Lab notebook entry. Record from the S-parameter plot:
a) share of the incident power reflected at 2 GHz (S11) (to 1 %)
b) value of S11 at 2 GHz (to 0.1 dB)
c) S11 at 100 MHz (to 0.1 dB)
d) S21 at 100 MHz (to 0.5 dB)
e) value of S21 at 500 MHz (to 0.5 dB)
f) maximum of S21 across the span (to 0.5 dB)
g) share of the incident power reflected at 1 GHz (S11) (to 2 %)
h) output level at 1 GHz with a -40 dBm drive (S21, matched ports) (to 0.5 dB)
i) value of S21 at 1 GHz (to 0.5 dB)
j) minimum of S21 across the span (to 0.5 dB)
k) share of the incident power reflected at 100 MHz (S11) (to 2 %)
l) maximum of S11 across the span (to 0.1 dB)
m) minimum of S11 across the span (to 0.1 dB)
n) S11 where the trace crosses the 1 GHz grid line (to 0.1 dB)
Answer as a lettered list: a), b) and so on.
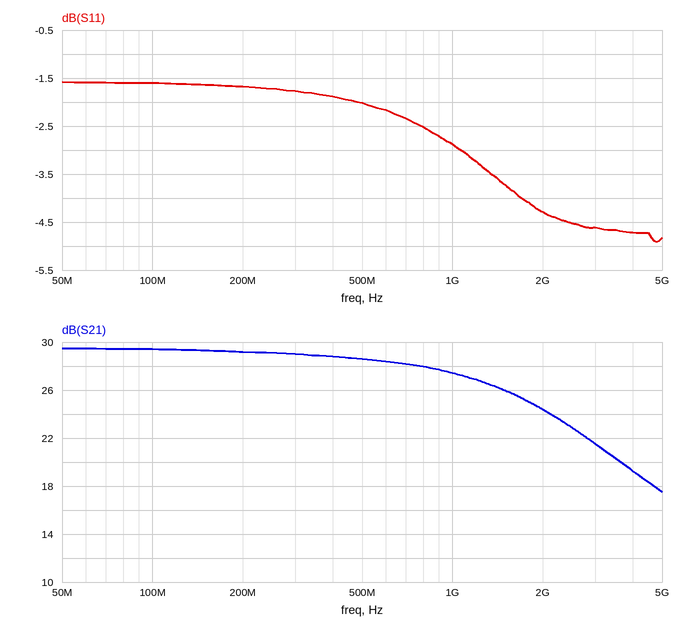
a) 37 %
b) -4.3 dB
c) -1.6 dB
d) 29.5 dB
e) 28.5 dB
f) 29.5 dB
g) 52 %
h) -12.5 dBm
i) 27.5 dB
j) 17.5 dB
k) 70 %
l) -1.6 dB
m) -4.9 dB
n) -2.9 dB
